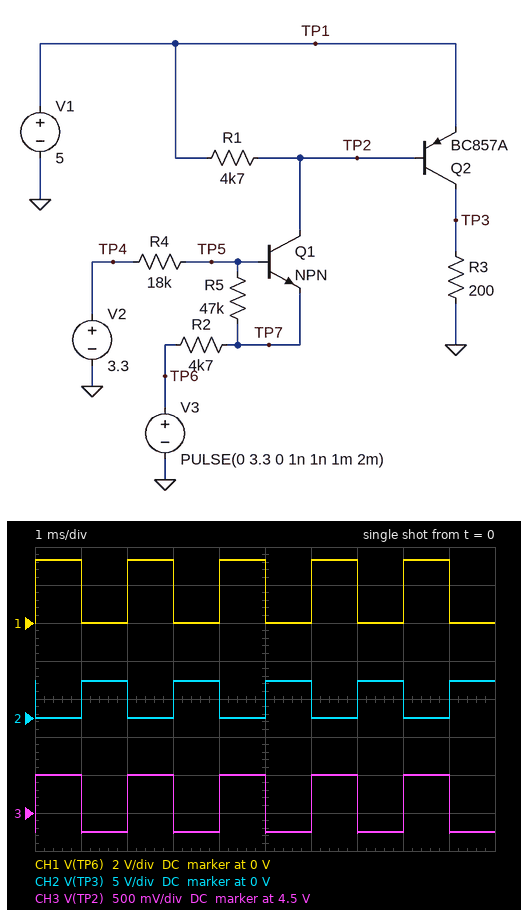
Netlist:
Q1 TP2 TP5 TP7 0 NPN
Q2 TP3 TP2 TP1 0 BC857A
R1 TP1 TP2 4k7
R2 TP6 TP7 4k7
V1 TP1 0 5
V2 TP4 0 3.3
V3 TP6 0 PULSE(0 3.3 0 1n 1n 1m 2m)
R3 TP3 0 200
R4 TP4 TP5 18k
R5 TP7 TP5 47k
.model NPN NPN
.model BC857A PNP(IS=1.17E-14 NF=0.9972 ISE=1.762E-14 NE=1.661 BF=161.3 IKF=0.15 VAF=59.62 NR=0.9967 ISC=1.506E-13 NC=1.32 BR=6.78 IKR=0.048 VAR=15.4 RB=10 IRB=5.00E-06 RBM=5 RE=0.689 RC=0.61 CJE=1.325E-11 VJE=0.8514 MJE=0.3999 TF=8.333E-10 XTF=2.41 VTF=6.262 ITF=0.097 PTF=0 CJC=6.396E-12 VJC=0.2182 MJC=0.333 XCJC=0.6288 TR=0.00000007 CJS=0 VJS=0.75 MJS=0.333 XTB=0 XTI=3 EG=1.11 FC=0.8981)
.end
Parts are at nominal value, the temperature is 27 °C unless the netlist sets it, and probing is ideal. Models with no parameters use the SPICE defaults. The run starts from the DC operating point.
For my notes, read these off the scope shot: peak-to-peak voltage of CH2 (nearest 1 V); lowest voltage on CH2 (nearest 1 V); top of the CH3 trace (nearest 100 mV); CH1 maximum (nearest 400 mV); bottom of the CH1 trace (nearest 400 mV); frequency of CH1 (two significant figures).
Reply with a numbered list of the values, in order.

1. 5 V
2. 0 V
3. 5.0 V
4. 3.2 V
5. 0 V
6. 500 Hz
